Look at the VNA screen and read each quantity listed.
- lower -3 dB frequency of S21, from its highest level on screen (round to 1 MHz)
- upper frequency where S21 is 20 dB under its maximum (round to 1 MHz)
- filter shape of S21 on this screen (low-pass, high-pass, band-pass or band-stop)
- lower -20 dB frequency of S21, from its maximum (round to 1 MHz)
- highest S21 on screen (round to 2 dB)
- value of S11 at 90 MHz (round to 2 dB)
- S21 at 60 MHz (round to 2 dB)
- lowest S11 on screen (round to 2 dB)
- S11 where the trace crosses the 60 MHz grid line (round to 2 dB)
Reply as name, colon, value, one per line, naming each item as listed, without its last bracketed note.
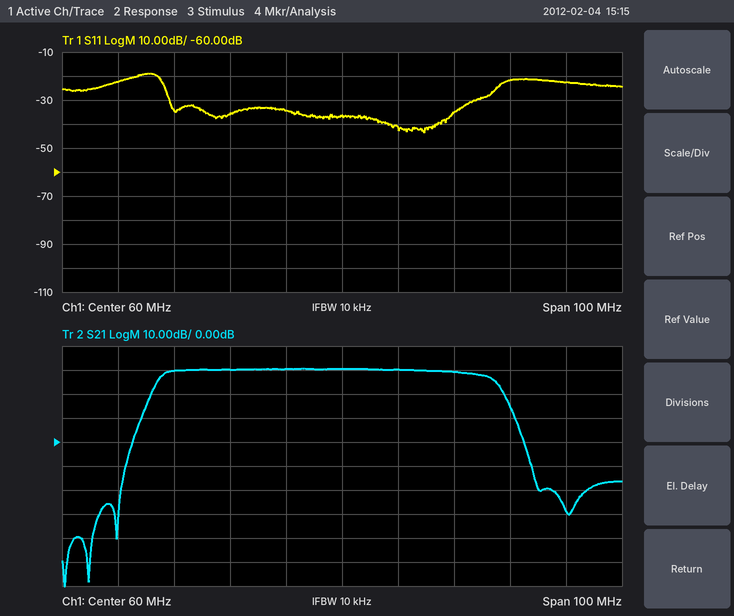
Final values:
lower -3 dB frequency of S21, from its highest level on screen: 28 MHz
upper frequency where S21 is 20 dB under its maximum: 91 MHz
filter shape of S21 on this screen: band-pass
lower -20 dB frequency of S21, from its maximum: 24 MHz
highest S21 on screen: 30 dB
value of S11 at 90 MHz: -22 dB
S21 at 60 MHz: 30 dB
lowest S11 on screen: -44 dB
S11 where the trace crosses the 60 MHz grid line: -36 dB
